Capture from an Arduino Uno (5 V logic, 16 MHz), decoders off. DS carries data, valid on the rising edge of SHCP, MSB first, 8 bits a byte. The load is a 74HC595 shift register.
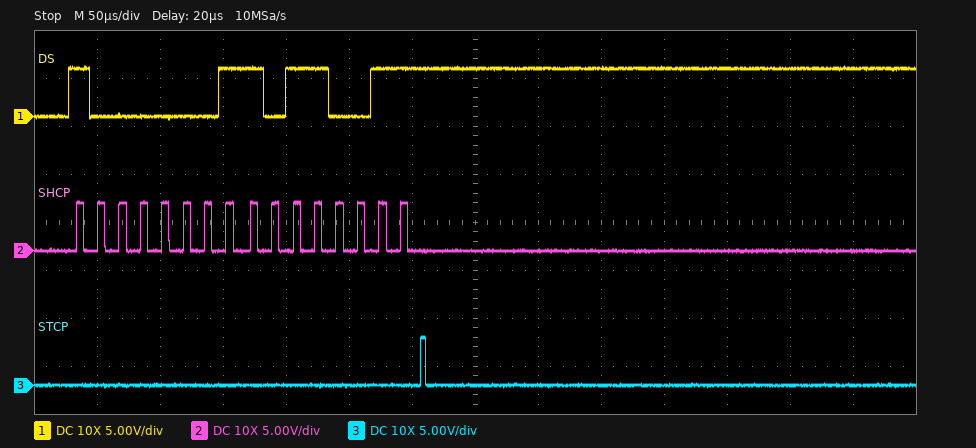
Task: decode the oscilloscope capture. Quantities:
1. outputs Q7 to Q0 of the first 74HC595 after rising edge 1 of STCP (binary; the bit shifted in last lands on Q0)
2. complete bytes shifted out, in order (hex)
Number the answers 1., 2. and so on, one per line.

1. 10110011
2. 81 B3
